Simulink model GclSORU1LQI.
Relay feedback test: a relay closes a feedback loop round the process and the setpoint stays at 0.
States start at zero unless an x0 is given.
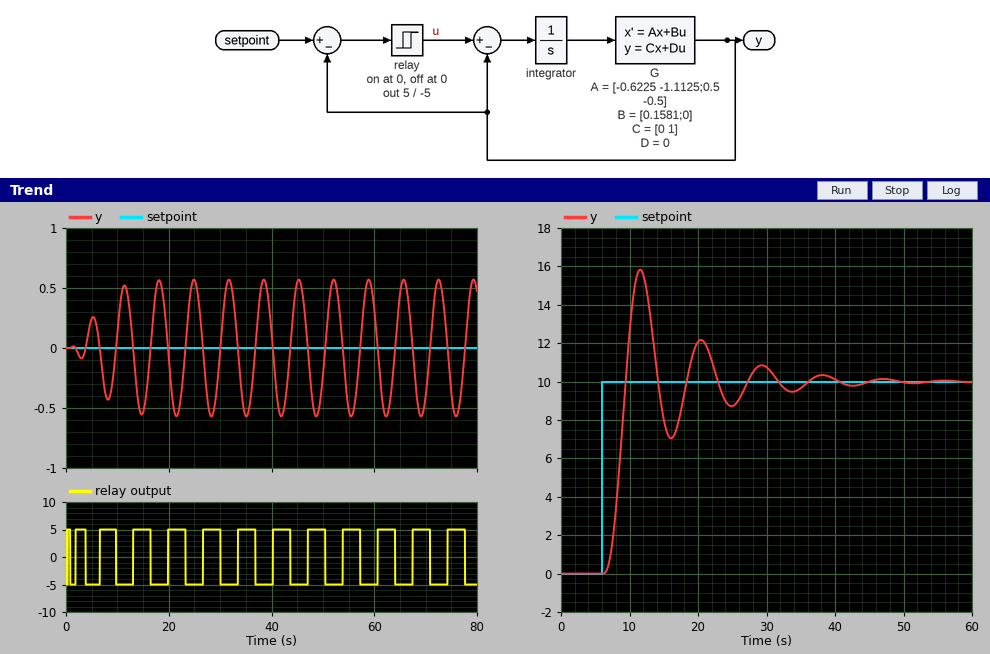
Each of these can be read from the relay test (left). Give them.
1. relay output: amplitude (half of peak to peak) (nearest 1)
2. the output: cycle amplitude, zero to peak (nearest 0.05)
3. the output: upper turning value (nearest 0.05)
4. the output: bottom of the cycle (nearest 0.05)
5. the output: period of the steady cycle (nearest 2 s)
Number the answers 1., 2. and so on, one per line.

1. 5
2. 0.55
3. 0.55
4. -0.55
5. 6 s
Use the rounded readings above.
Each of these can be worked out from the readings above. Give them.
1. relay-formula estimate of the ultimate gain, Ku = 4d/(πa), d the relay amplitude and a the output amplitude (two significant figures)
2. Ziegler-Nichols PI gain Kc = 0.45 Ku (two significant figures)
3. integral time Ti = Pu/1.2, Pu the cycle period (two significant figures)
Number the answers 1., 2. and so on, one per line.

1. 12
2. 5.4
3. 5.0 s
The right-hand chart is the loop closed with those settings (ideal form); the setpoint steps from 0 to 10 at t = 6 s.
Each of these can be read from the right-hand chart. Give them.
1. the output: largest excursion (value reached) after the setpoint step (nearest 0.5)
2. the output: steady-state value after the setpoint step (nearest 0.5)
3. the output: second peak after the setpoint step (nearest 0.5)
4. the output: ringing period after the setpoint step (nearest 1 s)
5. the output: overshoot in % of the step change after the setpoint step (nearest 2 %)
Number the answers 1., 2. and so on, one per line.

1. 16.0
2. 10.0
3. 12.0
4. 9 s
5. 58 %
